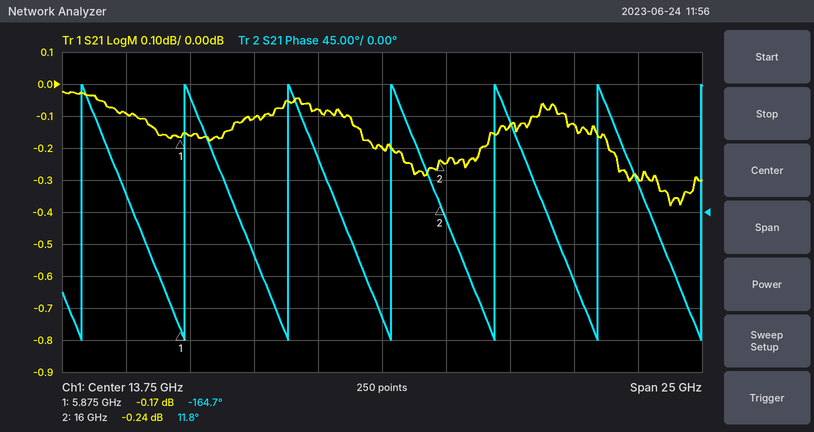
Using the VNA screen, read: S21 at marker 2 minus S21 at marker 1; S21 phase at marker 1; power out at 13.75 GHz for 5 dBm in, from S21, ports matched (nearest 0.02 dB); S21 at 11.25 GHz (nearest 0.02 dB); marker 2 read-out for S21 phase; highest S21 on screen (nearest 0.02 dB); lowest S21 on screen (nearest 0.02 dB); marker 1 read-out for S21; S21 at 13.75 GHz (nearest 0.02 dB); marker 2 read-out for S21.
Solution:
-0.07 dB
-164.7°
4.80 dBm
-0.08 dB
11.8°
-0.02 dB
-0.38 dB
-0.17 dB
-0.20 dB
-0.24 dB
